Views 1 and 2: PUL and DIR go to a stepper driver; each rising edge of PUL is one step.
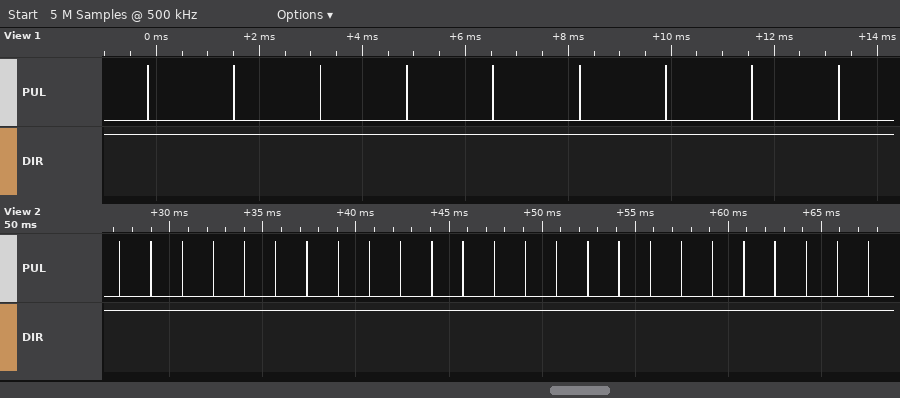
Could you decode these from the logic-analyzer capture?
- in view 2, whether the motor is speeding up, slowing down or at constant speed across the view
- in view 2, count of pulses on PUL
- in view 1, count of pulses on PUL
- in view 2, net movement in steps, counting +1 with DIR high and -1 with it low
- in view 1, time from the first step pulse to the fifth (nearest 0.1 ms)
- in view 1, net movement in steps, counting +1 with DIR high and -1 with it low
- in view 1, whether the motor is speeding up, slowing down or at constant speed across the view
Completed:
constant speed
25
9
+25
6.7 ms
+9
constant speed
